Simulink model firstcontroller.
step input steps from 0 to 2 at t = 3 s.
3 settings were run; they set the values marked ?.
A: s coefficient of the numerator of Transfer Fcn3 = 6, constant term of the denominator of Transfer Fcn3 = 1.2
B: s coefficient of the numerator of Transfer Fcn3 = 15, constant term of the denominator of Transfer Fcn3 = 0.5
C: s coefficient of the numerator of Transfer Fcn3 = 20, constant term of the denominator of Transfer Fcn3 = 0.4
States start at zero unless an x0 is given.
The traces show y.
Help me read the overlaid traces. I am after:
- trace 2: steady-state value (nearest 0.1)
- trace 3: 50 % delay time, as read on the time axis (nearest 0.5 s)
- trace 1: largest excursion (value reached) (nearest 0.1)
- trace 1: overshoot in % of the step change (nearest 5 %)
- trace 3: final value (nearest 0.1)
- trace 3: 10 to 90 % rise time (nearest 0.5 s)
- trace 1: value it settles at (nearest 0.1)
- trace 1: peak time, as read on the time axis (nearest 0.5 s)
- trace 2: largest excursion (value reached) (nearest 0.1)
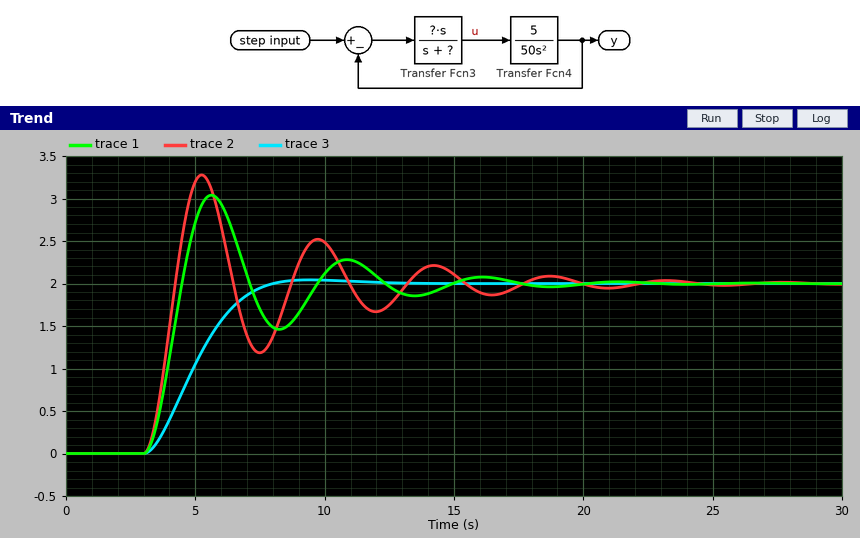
2.0
5.0 s
3.0
50 %
2.0
3.0 s
2.0
5.5 s
3.3
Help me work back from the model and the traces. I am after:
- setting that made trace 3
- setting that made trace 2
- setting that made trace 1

A
C
B
